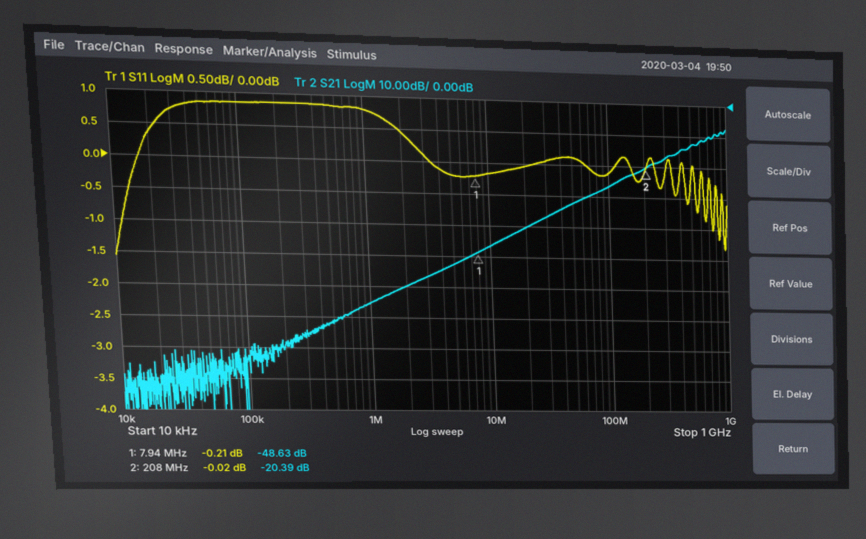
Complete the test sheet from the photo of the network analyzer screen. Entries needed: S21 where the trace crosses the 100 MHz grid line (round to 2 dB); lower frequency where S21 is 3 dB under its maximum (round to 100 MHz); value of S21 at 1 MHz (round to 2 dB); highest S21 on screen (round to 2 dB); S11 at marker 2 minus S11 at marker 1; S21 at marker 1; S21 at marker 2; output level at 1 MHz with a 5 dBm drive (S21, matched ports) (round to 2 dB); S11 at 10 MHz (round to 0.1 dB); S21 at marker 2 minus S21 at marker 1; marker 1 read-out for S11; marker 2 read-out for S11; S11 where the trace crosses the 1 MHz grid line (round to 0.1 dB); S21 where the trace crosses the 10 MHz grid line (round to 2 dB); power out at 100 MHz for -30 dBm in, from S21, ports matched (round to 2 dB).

-26 dB
700 MHz
-66 dB
-8 dB
0.19 dB
-48.63 dB
-20.39 dB
-60 dBm
-0.2 dB
28.24 dB
-0.21 dB
-0.02 dB
0.8 dB
-46 dB
-56 dBm
